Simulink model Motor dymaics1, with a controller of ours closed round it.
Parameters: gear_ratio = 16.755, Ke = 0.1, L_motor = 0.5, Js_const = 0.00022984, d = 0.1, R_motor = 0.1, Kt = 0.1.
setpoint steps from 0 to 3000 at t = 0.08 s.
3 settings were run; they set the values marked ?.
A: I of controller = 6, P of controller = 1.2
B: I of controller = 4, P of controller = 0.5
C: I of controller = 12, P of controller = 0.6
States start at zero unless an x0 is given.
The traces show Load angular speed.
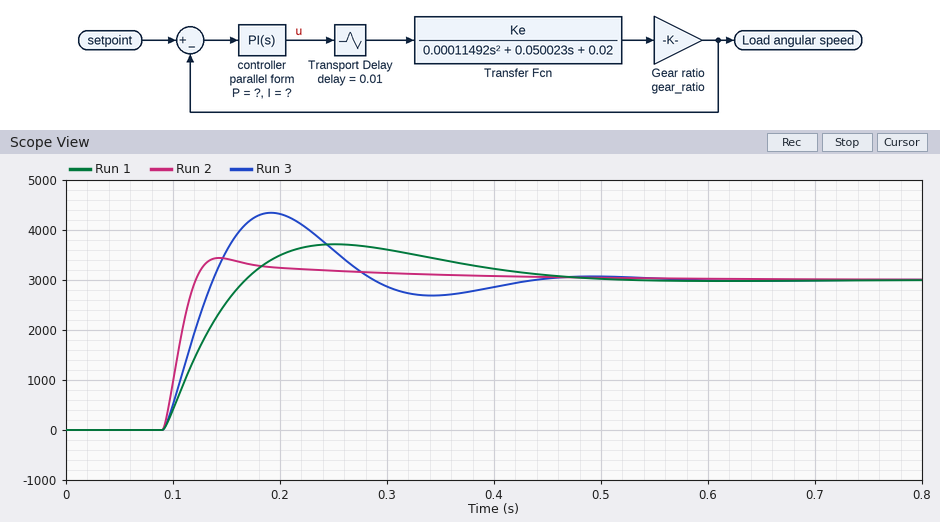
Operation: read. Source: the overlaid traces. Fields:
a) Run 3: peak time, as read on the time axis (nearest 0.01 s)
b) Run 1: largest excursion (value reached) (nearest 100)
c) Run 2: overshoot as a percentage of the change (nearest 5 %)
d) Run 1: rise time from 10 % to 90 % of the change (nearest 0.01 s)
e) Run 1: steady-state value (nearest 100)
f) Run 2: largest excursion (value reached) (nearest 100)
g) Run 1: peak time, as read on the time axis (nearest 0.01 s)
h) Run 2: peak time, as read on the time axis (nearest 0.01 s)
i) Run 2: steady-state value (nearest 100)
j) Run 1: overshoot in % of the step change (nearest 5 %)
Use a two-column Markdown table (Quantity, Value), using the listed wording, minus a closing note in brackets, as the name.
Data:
| Quantity | Value |
|---|---|
| Run 3: peak time, as read on the time axis | 0.19 s |
| Run 1: largest excursion (value reached) | 3700 |
| Run 2: overshoot as a percentage of the change | 15 % |
| Run 1: rise time from 10 % to 90 % of the change | 0.06 s |
| Run 1: steady-state value | 3000 |
| Run 2: largest excursion (value reached) | 3400 |
| Run 1: peak time, as read on the time axis | 0.25 s |
| Run 2: peak time, as read on the time axis | 0.14 s |
| Run 2: steady-state value | 3000 |
| Run 1: overshoot in % of the step change | 25 % |
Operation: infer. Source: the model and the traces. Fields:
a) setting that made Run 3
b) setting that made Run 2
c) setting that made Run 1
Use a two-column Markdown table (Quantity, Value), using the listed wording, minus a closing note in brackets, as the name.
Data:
| Quantity | Value |
|---|---|
| setting that made Run 3 | C |
| setting that made Run 2 | A |
| setting that made Run 1 | B |
